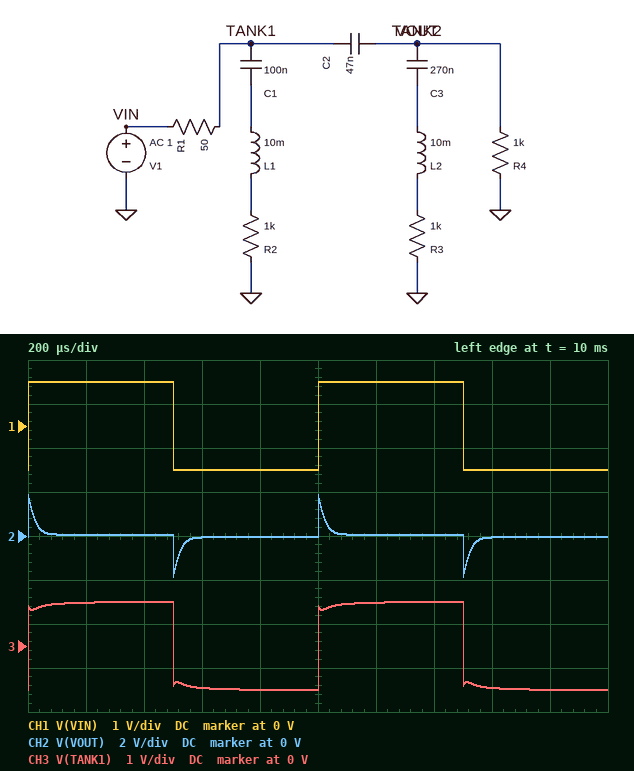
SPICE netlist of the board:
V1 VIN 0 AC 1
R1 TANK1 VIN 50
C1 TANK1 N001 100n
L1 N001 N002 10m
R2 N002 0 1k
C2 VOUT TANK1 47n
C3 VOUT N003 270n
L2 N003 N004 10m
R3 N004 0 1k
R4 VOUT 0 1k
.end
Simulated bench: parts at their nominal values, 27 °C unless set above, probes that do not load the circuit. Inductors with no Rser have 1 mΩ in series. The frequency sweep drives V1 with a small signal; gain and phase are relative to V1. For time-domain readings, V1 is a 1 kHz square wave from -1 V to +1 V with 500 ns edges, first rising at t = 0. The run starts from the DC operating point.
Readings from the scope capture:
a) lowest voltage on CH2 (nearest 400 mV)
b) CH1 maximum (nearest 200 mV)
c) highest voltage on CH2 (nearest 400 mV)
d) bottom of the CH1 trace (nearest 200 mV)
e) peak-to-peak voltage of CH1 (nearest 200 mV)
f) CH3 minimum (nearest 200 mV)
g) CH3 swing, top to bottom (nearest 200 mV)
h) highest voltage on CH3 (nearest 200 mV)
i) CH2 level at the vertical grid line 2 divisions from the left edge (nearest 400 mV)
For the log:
-2.0 V
1.0 V
2.0 V
-1.0 V
2.0 V
-1.0 V
2.0 V
1.0 V
0 V
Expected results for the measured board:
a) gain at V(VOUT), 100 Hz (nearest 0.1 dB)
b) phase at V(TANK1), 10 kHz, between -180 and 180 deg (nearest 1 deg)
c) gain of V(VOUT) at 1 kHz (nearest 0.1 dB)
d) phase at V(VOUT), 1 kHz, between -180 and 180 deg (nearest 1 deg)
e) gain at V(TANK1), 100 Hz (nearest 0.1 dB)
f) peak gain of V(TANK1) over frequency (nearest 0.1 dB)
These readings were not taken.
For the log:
-31.0 dB
-1 deg
-16.4 dB
66 deg
0 dB
0 dB
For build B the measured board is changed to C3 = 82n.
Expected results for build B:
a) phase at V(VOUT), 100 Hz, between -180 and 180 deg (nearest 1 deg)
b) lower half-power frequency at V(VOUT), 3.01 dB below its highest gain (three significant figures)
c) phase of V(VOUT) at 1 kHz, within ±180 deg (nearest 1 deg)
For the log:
85 deg
7.00 kHz
58 deg
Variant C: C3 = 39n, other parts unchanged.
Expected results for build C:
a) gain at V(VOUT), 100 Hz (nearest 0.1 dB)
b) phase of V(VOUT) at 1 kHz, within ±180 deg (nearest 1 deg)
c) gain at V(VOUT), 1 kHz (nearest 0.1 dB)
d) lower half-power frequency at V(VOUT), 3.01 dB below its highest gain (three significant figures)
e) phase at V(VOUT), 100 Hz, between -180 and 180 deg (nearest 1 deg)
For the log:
-30.6 dB
61 deg
-12.2 dB
7.84 kHz
87 deg
